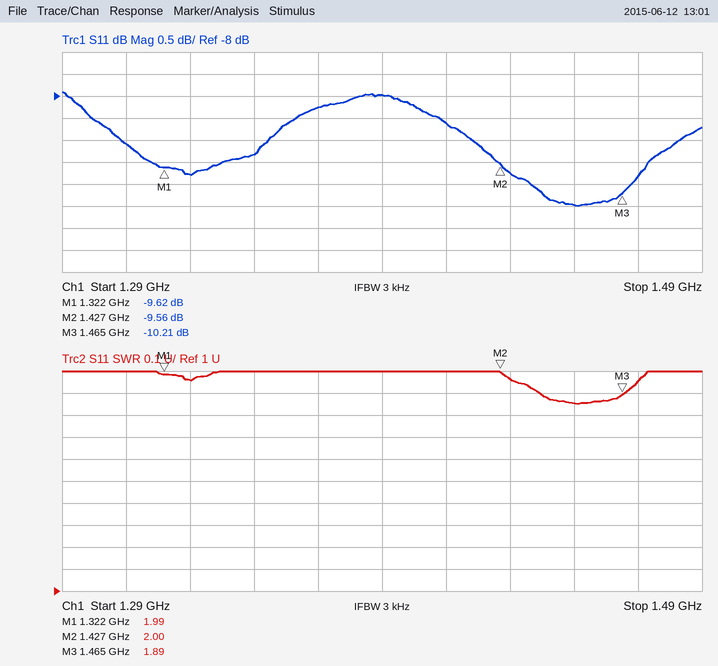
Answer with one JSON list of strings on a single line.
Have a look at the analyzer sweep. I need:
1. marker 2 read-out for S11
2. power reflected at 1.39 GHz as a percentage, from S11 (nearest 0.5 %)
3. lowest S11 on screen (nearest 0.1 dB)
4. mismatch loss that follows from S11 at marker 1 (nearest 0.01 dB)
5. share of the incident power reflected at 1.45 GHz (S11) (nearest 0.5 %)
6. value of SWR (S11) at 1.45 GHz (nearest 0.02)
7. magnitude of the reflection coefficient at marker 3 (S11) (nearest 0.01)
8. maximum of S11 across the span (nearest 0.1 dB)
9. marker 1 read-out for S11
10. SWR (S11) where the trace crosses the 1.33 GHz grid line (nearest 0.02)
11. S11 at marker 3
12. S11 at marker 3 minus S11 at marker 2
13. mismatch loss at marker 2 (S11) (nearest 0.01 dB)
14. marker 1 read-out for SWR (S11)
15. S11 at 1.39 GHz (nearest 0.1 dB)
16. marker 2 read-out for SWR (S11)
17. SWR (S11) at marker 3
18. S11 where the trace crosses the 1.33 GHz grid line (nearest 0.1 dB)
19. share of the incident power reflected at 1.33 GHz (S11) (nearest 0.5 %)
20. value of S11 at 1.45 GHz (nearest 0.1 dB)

["-9.56 dB", "16.0 %", "-10.5 dB", "0.50 dB", "9.0 %", "1.86", "0.31", "-7.9 dB", "-9.62 dB", "1.96", "-10.21 dB", "-0.65 dB", "0.51 dB", "1.99", "-8.0 dB", "2.00", "1.89", "-9.8 dB", "10.5 %", "-10.5 dB"]
